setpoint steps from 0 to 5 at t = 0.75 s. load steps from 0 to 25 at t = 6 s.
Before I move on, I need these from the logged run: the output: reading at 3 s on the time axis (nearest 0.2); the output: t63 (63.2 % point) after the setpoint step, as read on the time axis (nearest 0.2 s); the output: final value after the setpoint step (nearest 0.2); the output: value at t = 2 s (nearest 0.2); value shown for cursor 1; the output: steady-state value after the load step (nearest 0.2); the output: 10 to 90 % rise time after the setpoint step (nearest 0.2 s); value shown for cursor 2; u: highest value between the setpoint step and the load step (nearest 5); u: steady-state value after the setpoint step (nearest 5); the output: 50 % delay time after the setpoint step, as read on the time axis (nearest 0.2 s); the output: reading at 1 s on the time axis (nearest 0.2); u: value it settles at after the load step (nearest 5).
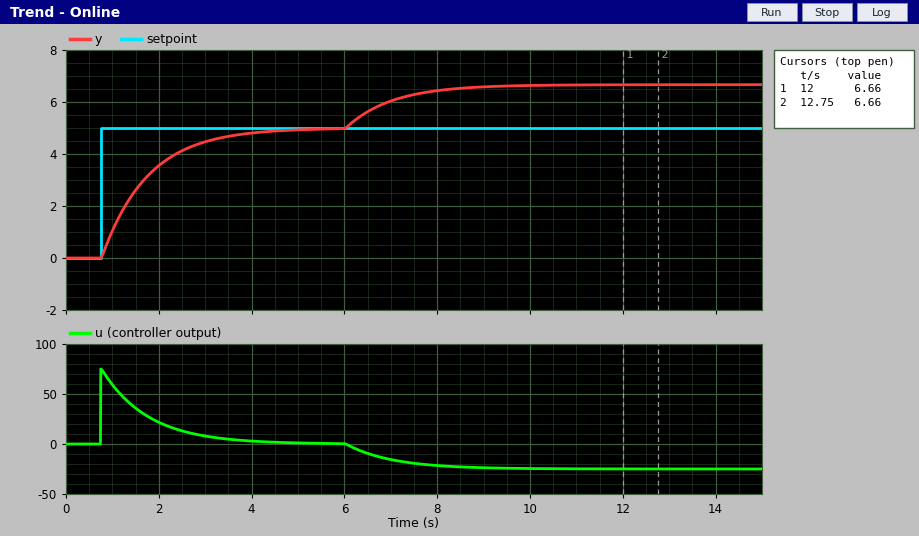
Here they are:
4.4
1.8 s
5.0
3.6
6.66
6.6
2.2 s
6.66
75
0
1.4 s
1.0
-25
